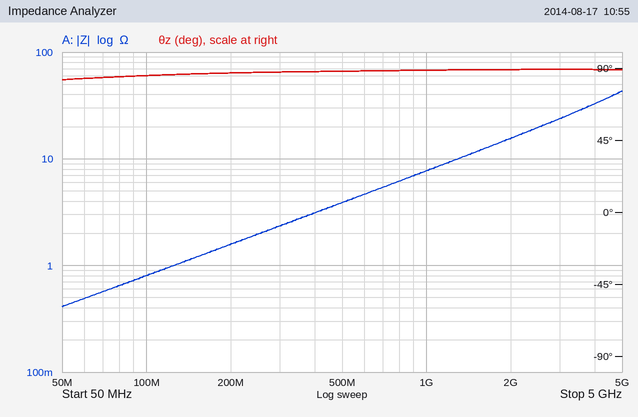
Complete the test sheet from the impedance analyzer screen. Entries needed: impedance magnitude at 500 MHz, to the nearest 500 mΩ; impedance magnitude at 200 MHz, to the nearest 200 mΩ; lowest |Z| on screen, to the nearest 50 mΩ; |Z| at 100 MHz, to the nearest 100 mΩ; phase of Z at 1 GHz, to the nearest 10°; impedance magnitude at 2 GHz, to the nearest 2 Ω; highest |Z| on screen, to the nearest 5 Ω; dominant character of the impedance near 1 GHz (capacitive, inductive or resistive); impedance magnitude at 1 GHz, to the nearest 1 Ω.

4.0 Ω
1.6 Ω
400 mΩ
800 mΩ
90°
16 Ω
45 Ω
inductive
8 Ω
